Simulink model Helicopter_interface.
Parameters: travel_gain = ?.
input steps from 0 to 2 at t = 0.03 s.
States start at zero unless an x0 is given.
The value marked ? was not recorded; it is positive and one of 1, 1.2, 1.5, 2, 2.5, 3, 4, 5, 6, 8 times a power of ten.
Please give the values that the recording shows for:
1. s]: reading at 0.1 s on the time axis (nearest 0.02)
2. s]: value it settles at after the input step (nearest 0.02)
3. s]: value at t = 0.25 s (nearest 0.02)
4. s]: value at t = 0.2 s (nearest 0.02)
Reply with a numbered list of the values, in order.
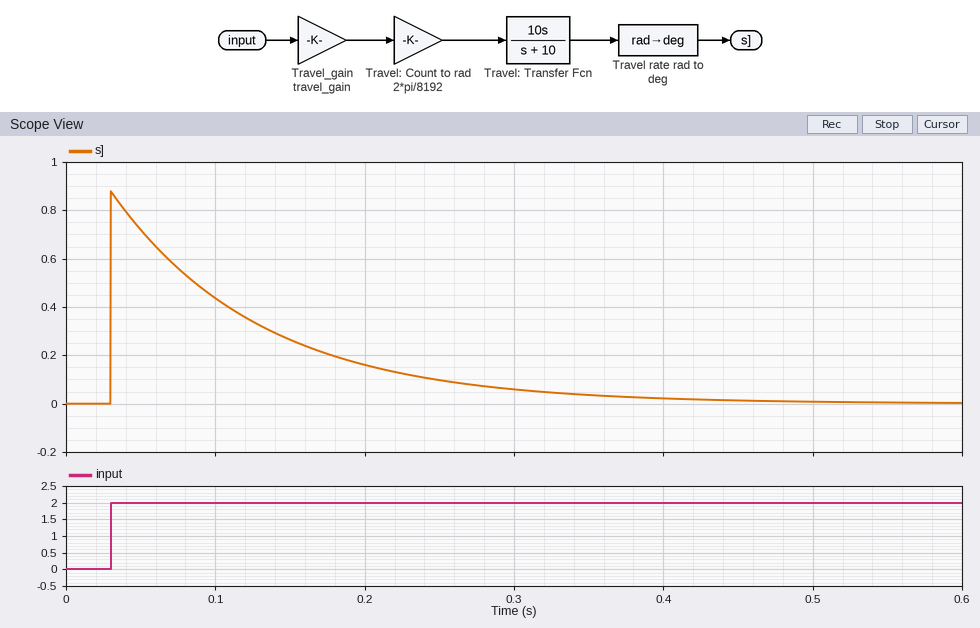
1. 0.44
2. 0.00
3. 0.10
4. 0.16
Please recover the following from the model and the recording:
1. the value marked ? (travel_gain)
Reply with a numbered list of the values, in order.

1. 1
